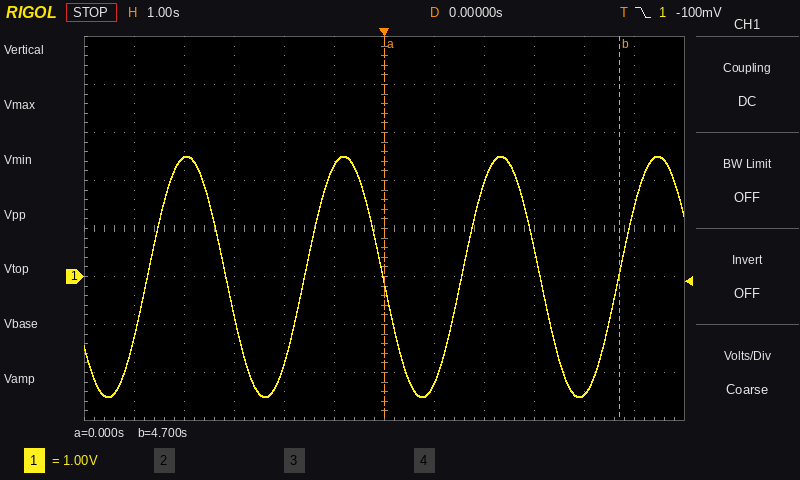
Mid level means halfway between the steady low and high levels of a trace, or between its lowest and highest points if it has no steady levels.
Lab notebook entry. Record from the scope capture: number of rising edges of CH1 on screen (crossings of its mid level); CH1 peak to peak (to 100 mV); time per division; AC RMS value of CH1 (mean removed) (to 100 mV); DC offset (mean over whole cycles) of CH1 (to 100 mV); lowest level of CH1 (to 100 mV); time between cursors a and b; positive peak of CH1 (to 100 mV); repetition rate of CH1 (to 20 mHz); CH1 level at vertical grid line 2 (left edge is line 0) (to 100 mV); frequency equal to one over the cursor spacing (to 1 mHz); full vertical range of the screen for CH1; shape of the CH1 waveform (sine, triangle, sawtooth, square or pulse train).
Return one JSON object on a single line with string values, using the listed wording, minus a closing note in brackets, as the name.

{"number of rising edges of CH1 on screen": "4", "CH1 peak to peak": "5.0 V", "time per division": "1 s", "AC RMS value of CH1 (mean removed)": "1.8 V", "DC offset (mean over whole cycles) of CH1": "0.0 V", "lowest level of CH1": "-2.5 V", "time between cursors a and b": "4.7 s", "positive peak of CH1": "2.5 V", "repetition rate of CH1": "320 mHz", "CH1 level at vertical grid line 2 (left edge is line 0)": "2.5 V", "frequency equal to one over the cursor spacing": "213 mHz", "full vertical range of the screen for CH1": "8 V", "shape of the CH1 waveform": "sine"}
